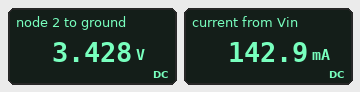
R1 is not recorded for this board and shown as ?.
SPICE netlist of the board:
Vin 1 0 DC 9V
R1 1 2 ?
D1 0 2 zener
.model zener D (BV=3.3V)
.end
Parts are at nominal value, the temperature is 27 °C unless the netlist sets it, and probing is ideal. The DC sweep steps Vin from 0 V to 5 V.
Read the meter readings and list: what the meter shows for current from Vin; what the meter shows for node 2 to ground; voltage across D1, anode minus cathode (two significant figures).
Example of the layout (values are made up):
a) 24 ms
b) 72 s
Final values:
a) 142.9 mA
b) 3.428 V
c) -3.4 V
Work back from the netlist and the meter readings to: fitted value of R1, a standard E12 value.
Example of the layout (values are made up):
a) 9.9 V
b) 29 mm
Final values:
a) 39 Ω
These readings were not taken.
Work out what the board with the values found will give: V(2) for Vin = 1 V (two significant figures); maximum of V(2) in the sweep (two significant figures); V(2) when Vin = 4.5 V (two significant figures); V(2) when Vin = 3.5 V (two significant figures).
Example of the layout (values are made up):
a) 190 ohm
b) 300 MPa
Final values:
a) 1.0 V
b) 3.4 V
c) 3.4 V
d) 3.3 V
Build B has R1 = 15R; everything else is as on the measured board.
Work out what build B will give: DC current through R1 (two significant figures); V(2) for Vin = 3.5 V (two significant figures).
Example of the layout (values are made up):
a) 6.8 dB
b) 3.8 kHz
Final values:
a) 370 mA
b) 3.4 V
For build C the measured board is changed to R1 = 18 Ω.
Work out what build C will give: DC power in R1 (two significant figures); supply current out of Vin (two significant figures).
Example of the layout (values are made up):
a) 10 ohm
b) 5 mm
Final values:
a) 1.7 W
b) 310 mA
